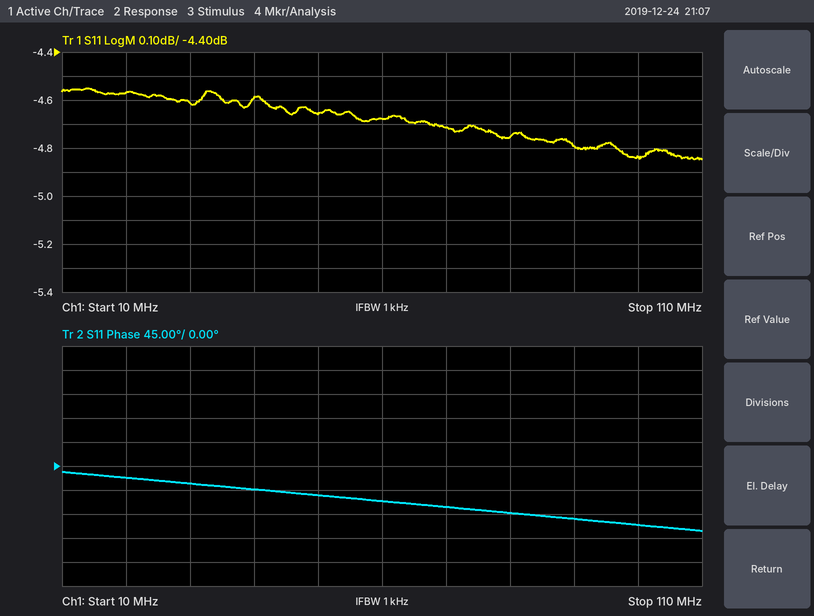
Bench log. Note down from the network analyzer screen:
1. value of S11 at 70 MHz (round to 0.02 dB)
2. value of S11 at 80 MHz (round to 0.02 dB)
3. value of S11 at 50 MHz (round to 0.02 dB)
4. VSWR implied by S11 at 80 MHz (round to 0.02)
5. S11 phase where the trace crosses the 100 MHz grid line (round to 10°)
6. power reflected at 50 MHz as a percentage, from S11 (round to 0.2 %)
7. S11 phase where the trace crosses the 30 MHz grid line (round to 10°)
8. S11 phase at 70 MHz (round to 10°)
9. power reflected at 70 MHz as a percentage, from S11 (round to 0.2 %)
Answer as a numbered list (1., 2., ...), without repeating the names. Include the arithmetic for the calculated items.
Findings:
1. -4.72 dB
2. -4.76 dB
3. -4.66 dB
4. |Γ| = 10^(-4.76/20) = 0.5781; VSWR = (1 + 0.5781)/(1 − 0.5781) ≈ 3.74
5. -110°
6. 10^(-4.66/10) ≈ 34.2 %
7. -30°
8. -80°
9. 10^(-4.72/10) ≈ 33.7 %, so 33.8 % to the nearest 0.2 %
